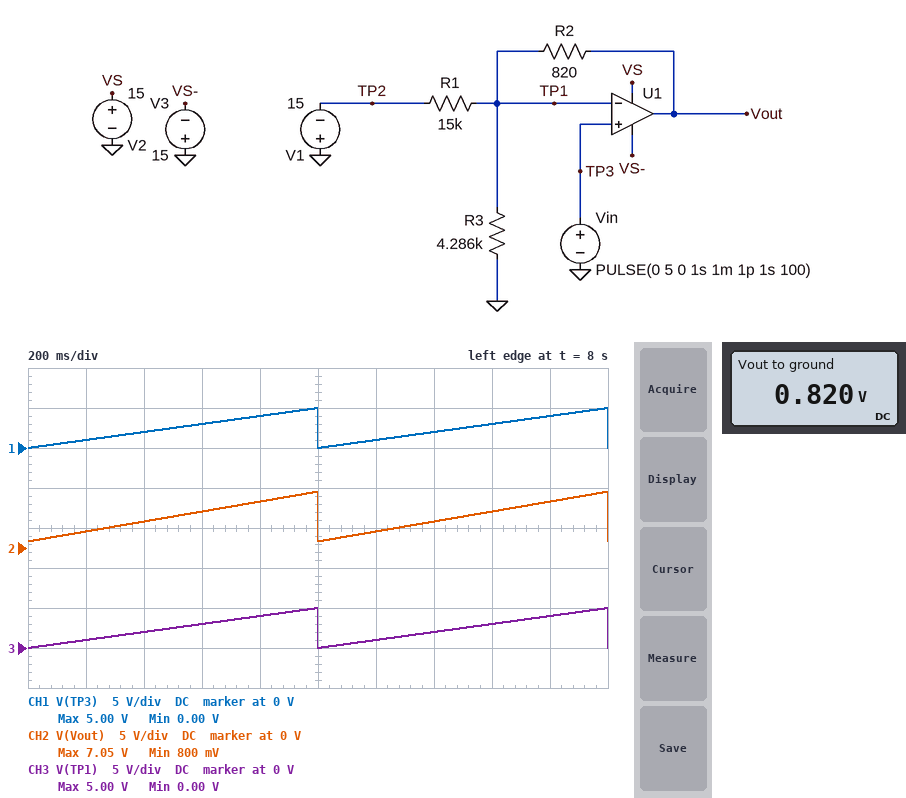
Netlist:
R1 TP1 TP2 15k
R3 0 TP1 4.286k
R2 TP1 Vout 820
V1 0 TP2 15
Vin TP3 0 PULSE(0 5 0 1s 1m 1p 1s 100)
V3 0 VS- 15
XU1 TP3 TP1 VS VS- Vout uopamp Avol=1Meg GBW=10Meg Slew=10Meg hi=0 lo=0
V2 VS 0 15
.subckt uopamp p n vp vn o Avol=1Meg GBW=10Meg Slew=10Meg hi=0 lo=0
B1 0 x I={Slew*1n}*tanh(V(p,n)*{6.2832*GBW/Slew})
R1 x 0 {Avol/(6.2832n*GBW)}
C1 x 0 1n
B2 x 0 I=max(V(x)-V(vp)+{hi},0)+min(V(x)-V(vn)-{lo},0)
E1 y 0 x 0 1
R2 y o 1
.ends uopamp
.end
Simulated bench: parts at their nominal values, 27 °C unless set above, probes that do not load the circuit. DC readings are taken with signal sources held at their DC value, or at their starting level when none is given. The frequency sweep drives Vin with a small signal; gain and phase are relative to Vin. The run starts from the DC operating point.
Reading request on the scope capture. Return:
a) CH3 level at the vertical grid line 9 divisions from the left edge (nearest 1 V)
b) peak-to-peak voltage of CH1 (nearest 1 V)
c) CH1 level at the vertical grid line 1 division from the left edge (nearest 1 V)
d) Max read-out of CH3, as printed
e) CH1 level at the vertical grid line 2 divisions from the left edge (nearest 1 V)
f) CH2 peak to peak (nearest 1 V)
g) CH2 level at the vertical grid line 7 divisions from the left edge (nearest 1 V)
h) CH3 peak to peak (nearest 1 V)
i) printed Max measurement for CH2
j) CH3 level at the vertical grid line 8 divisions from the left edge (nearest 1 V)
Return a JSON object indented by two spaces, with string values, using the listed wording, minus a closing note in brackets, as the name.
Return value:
{
  "CH3 level at the vertical grid line 9 divisions from the left edge": "4 V",
  "peak-to-peak voltage of CH1": "5 V",
  "CH1 level at the vertical grid line 1 division from the left edge": "1 V",
  "Max read-out of CH3, as printed": "5.00 V",
  "CH1 level at the vertical grid line 2 divisions from the left edge": "2 V",
  "CH2 peak to peak": "6 V",
  "CH2 level at the vertical grid line 7 divisions from the left edge": "3 V",
  "CH3 peak to peak": "5 V",
  "printed Max measurement for CH2": "7.05 V",
  "CH3 level at the vertical grid line 8 divisions from the left edge": "3 V"
}
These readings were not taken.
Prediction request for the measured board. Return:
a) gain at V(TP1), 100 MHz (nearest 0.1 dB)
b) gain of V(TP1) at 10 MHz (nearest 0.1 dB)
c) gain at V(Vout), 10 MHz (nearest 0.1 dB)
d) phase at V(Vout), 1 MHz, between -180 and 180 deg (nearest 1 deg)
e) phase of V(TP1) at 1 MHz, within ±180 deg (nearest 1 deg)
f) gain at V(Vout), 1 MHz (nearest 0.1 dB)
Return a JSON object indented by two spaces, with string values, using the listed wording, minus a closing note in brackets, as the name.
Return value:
{
  "gain at V(TP1), 100 MHz": "-21.9 dB",
  "gain of V(TP1) at 10 MHz": "-4.1 dB",
  "gain at V(Vout), 10 MHz": "-2.2 dB",
  "phase at V(Vout), 1 MHz, between -180 and 180 deg": "-7 deg",
  "phase of V(TP1) at 1 MHz, within ±180 deg": "-7 deg",
  "gain at V(Vout), 1 MHz": "1.8 dB"
}
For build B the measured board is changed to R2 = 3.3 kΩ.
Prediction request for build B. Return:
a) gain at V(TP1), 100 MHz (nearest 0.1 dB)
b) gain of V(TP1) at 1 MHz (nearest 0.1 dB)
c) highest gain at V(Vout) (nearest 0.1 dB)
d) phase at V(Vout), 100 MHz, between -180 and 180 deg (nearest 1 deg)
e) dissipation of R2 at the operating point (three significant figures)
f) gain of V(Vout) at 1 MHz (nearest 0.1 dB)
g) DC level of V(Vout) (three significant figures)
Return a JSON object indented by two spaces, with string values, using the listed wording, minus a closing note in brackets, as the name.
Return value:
{
  "gain at V(TP1), 100 MHz": "-26.0 dB",
  "gain of V(TP1) at 1 MHz": "-0.2 dB",
  "highest gain at V(Vout)": "6.0 dB",
  "phase at V(Vout), 100 MHz, between -180 and 180 deg": "-87 deg",
  "dissipation of R2 at the operating point": "3.30 mW",
  "gain of V(Vout) at 1 MHz": "5.8 dB",
  "DC level of V(Vout)": "3.30 V"
}
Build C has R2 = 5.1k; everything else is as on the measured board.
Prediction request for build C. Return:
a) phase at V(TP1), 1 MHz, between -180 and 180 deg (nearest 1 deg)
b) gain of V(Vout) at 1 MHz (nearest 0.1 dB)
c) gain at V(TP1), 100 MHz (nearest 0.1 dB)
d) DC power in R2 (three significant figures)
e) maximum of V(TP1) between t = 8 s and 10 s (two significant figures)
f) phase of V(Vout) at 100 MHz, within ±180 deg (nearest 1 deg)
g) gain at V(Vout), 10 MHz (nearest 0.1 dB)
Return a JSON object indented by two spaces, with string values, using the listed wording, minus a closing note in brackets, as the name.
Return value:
{
  "phase at V(TP1), 1 MHz, between -180 and 180 deg": "-14 deg",
  "gain of V(Vout) at 1 MHz": "7.8 dB",
  "gain at V(TP1), 100 MHz": "-28.1 dB",
  "DC power in R2": "5.10 mW",
  "maximum of V(TP1) between t = 8 s and 10 s": "3.9 V",
  "phase of V(Vout) at 100 MHz, within ±180 deg": "-88 deg",
  "gain at V(Vout), 10 MHz": "-0.6 dB"
}
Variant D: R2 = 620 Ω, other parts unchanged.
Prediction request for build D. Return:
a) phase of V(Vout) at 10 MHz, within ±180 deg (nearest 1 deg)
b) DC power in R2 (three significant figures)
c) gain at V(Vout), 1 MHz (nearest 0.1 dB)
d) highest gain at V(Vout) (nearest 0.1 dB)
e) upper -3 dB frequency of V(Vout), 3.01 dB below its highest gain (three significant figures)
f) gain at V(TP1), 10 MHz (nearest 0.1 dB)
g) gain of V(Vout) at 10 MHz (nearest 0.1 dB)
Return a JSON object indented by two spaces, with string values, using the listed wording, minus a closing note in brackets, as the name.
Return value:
{
  "phase of V(Vout) at 10 MHz, within ±180 deg": "-50 deg",
  "DC power in R2": "620 µW",
  "gain at V(Vout), 1 MHz": "1.4 dB",
  "highest gain at V(Vout)": "1.5 dB",
  "upper -3 dB frequency of V(Vout), 3.01 dB below its highest gain": "8.43 MHz",
  "gain at V(TP1), 10 MHz": "-3.8 dB",
  "gain of V(Vout) at 10 MHz": "-2.3 dB"
}
